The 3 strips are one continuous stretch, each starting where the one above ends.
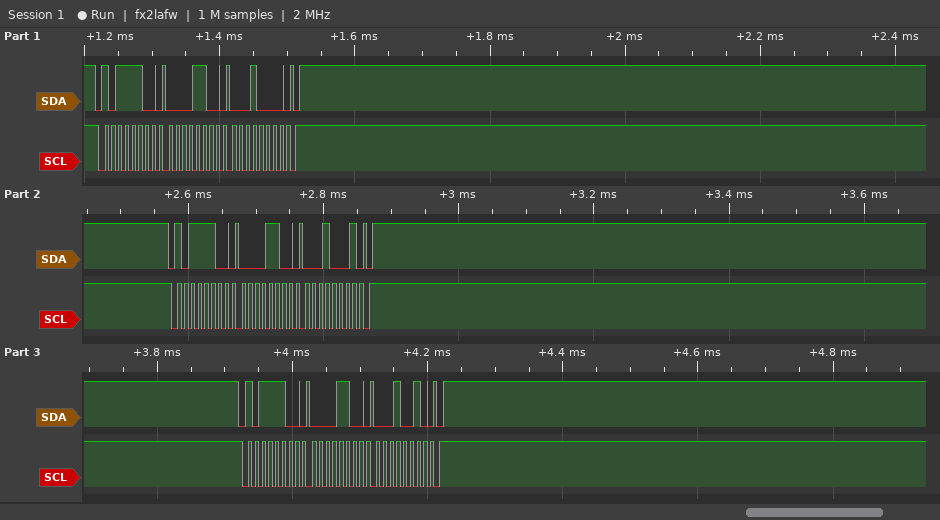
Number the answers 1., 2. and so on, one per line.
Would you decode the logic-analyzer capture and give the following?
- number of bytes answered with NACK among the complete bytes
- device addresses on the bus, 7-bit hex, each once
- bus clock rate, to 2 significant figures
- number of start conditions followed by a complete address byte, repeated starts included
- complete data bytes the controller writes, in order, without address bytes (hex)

1. 0
2. 0x5E
3. 100 kHz
4. 3
5. 0C 10 0C 11 0C 12
